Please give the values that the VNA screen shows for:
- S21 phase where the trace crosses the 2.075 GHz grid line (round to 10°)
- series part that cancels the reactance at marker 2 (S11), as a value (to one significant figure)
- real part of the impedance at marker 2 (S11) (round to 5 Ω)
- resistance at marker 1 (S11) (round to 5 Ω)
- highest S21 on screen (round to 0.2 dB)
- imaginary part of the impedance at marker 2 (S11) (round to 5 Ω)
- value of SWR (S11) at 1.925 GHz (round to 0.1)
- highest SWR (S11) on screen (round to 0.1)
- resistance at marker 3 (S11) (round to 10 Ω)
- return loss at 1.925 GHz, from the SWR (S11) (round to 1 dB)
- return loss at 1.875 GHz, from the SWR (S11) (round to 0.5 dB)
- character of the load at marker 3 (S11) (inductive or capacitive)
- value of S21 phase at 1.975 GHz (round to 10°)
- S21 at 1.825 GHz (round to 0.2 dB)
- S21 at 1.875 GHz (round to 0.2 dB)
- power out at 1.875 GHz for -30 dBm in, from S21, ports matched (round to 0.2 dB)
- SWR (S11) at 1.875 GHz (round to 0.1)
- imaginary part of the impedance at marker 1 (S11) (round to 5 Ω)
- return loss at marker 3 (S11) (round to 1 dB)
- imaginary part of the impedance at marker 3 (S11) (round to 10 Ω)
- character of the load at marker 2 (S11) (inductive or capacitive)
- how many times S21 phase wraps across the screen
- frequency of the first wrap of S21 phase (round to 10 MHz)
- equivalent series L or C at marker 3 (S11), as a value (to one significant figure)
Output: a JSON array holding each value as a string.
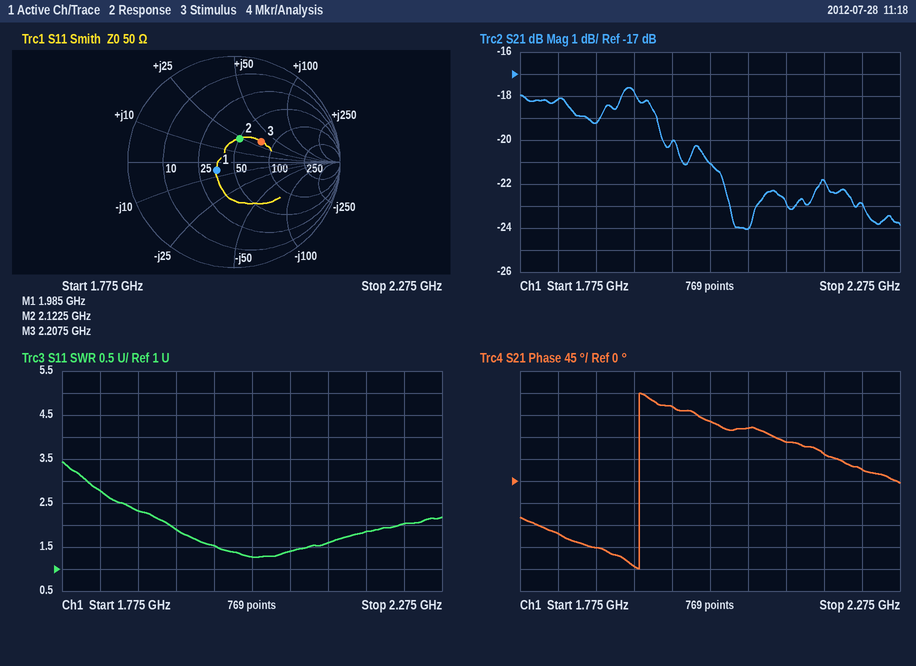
["110°", "3 pF", "50 Ω", "35 Ω", "-17.6 dB", "+25 Ω", "1.9", "3.4", "80 Ω", "10 dB", "8.0 dB", "inductive", "150°", "-18.2 dB", "-19.2 dB", "-49.2 dBm", "2.3", "-5 Ω", "10 dB", "+30 Ω", "inductive", "1", "1.93 GHz", "2 nH"]
